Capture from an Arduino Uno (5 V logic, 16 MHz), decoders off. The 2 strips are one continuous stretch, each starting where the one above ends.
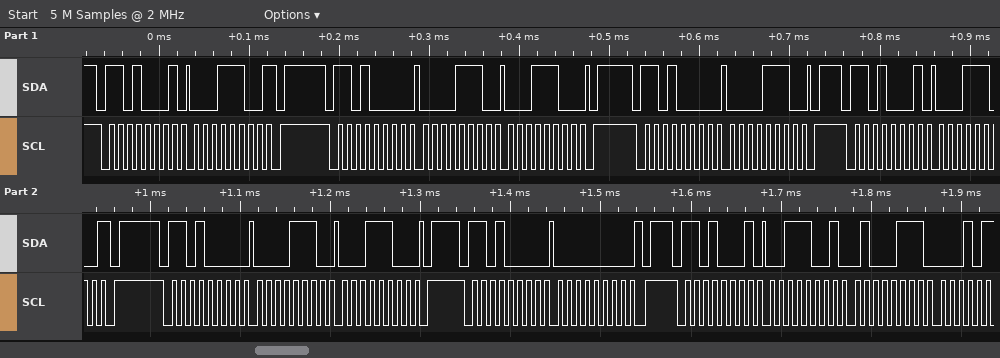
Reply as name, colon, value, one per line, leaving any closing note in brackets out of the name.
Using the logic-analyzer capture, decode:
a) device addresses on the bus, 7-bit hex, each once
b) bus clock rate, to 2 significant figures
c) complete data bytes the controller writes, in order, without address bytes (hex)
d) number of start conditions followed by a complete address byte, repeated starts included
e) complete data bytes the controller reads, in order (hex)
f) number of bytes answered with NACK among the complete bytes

device addresses on the bus, 7-bit hex, each once: 0x68
bus clock rate, to 2 significant figures: 100 kHz
complete data bytes the controller writes, in order, without address bytes: 0E 1C 0E 0E 1C 00
number of start conditions followed by a complete address byte, repeated starts included: 7
complete data bytes the controller reads, in order: 1C 1C 39 47
number of bytes answered with NACK among the complete bytes: 2
